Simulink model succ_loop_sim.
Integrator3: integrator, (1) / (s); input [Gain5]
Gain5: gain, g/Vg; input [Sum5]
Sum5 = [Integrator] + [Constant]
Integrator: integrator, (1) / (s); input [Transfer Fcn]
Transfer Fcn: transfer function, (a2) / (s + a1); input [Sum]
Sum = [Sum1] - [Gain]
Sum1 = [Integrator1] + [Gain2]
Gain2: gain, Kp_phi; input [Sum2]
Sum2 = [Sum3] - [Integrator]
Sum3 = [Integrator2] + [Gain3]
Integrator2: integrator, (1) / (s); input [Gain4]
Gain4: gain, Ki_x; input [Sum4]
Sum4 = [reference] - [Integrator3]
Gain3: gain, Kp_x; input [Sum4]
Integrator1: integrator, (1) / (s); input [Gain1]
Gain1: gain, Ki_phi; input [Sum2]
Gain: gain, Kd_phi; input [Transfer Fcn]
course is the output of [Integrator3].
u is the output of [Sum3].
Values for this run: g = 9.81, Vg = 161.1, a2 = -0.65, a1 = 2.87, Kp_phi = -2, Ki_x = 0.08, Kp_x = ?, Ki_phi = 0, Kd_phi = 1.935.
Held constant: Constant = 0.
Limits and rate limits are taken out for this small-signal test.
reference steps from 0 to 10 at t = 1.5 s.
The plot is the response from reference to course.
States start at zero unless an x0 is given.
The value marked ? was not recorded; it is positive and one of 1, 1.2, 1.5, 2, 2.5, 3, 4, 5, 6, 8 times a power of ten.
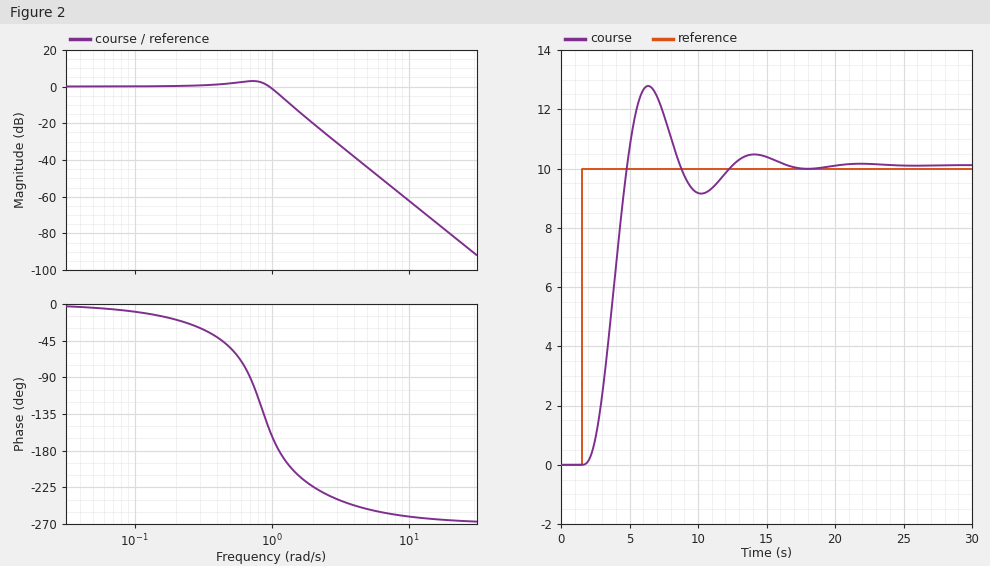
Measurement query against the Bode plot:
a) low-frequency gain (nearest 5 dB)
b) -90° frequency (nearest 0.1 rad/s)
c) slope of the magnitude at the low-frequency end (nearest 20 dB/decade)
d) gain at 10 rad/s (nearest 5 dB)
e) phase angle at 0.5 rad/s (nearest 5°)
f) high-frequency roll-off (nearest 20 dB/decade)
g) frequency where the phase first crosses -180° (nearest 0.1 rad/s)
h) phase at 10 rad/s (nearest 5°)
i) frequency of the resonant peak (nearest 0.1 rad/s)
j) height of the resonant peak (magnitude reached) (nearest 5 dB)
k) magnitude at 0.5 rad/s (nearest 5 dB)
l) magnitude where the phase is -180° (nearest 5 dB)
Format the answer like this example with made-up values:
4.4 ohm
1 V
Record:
0 dB
0.7 rad/s
0 dB/decade
-60 dB
-55°
-60 dB/decade
1.1 rad/s
-260°
0.7 rad/s
5 dB
0 dB
-5 dB
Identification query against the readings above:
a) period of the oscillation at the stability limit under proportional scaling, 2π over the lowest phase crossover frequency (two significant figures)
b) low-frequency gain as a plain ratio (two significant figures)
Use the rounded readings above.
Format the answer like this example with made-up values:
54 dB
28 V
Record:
5.7 s
1.0
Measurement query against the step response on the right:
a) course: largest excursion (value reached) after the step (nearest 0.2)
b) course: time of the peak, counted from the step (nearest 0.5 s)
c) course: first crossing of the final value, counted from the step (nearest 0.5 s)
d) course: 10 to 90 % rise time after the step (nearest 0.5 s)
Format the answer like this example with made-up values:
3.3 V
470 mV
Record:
12.8
5.0 s
3.5 s
2.0 s
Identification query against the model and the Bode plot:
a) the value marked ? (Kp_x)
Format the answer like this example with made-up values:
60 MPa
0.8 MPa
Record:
10
